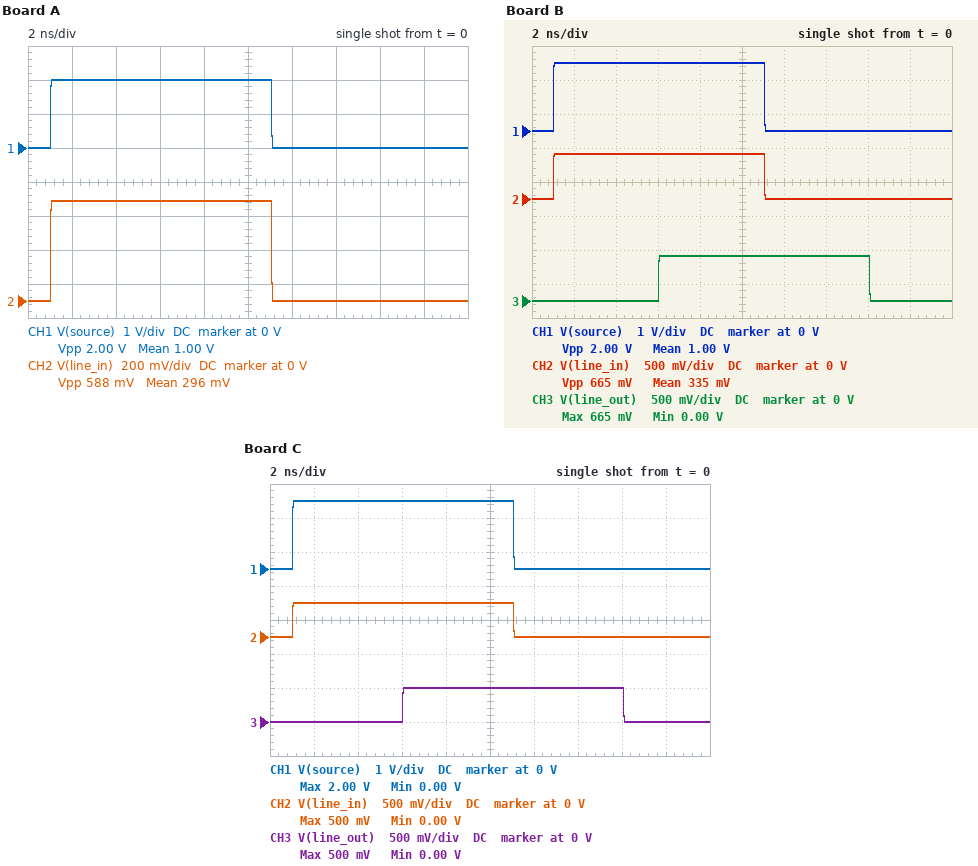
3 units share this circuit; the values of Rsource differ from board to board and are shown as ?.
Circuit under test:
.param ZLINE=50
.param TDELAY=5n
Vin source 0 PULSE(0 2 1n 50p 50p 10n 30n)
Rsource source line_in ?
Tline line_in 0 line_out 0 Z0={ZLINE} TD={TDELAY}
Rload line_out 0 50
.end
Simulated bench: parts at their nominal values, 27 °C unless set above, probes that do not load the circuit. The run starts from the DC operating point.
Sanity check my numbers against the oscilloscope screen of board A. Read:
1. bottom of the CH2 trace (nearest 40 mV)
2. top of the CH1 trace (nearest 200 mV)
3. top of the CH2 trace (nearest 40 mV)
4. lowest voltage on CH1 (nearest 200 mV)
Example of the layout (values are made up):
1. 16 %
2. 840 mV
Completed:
1. 0 V
2. 2.0 V
3. 600 mV
4. 0 V
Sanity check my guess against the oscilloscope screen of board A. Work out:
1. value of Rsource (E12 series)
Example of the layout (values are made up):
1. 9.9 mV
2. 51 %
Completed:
1. 120 Ω
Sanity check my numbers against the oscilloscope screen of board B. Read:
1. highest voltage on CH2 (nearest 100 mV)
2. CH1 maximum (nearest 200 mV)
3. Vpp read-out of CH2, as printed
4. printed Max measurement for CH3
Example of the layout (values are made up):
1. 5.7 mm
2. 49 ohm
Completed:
1. 700 mV
2. 2.0 V
3. 665 mV
4. 665 mV
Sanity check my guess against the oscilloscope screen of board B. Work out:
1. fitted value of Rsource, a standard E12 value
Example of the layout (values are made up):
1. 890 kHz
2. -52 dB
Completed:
1. 100 Ω
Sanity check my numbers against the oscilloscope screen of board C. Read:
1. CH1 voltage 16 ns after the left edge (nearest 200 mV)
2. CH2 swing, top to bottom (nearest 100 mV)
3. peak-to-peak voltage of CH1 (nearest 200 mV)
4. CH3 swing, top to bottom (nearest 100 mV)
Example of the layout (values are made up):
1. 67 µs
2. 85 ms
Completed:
1. 0 V
2. 500 mV
3. 2.0 V
4. 500 mV
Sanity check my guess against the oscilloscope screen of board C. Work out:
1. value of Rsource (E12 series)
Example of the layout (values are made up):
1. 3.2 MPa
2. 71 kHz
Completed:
1. 150 Ω
